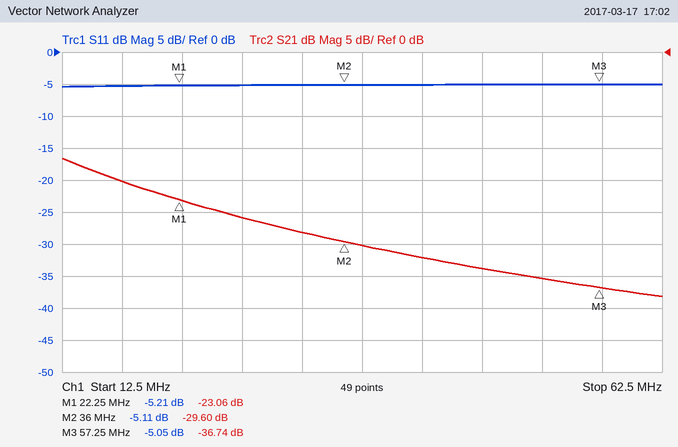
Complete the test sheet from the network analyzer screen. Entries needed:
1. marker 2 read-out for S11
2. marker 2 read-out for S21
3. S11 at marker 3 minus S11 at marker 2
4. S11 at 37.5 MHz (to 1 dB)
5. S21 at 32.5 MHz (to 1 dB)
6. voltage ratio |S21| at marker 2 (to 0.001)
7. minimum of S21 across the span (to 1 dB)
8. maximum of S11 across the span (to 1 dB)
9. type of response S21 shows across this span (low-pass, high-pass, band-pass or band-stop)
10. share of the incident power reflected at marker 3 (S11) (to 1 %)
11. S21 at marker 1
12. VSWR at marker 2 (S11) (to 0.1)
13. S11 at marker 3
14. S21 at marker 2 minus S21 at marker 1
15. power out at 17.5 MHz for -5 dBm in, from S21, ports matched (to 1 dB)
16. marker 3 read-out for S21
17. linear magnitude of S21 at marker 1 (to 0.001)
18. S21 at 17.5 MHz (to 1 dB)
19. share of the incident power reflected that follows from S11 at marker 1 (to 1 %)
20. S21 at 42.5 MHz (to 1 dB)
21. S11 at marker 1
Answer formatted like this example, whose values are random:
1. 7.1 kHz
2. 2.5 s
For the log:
1. -5.11 dB
2. -29.60 dB
3. 0.06 dB
4. -5 dB
5. -28 dB
6. 0.033
7. -38 dB
8. -5 dB
9. low-pass
10. 31 %
11. -23.06 dB
12. 3.5
13. -5.05 dB
14. -6.54 dB
15. -25 dBm
16. -36.74 dB
17. 0.070
18. -20 dB
19. 30 %
20. -32 dB
21. -5.21 dB
